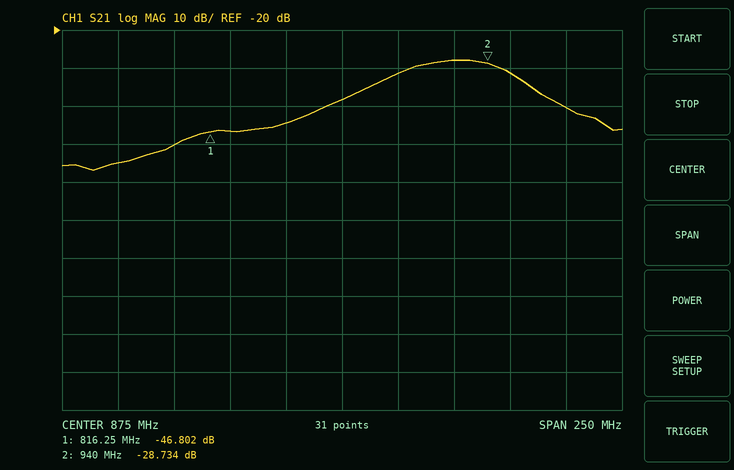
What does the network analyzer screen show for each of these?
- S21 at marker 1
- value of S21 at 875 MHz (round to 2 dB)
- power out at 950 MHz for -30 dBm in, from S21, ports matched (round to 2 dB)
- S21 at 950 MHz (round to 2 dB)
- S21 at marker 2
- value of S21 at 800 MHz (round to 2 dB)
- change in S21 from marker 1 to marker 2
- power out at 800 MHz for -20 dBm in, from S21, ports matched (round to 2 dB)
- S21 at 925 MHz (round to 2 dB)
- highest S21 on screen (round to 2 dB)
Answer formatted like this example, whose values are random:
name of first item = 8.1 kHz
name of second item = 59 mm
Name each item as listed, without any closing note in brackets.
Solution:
S21 at marker 1 = -46.802 dB
value of S21 at 875 MHz = -38 dB
power out at 950 MHz for -30 dBm in, from S21, ports matched = -62 dBm
S21 at 950 MHz = -32 dB
S21 at marker 2 = -28.734 dB
value of S21 at 800 MHz = -50 dB
change in S21 from marker 1 to marker 2 = 18.068 dB
power out at 800 MHz for -20 dBm in, from S21, ports matched = -70 dBm
S21 at 925 MHz = -28 dB
highest S21 on screen = -28 dB
